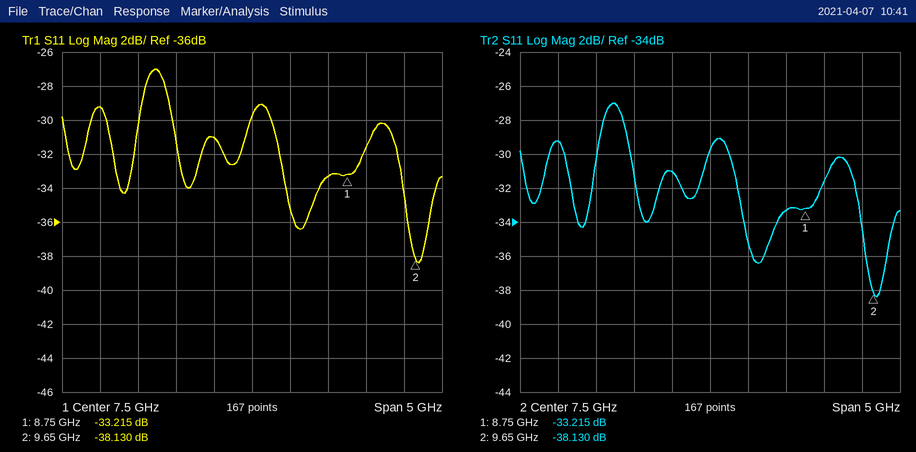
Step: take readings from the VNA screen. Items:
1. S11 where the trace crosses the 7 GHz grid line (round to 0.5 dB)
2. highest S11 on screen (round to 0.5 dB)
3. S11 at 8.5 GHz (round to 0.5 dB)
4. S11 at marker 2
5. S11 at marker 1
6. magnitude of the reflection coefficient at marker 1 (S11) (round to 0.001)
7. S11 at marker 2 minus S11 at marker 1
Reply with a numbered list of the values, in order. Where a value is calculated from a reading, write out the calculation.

1. -31.0 dB
2. -27.0 dB
3. -33.5 dB
4. -38.130 dB
5. -33.215 dB
6. 10^(-33.215/20) ≈ 0.022
7. -38.13 − (-33.215) = -4.915 dB
